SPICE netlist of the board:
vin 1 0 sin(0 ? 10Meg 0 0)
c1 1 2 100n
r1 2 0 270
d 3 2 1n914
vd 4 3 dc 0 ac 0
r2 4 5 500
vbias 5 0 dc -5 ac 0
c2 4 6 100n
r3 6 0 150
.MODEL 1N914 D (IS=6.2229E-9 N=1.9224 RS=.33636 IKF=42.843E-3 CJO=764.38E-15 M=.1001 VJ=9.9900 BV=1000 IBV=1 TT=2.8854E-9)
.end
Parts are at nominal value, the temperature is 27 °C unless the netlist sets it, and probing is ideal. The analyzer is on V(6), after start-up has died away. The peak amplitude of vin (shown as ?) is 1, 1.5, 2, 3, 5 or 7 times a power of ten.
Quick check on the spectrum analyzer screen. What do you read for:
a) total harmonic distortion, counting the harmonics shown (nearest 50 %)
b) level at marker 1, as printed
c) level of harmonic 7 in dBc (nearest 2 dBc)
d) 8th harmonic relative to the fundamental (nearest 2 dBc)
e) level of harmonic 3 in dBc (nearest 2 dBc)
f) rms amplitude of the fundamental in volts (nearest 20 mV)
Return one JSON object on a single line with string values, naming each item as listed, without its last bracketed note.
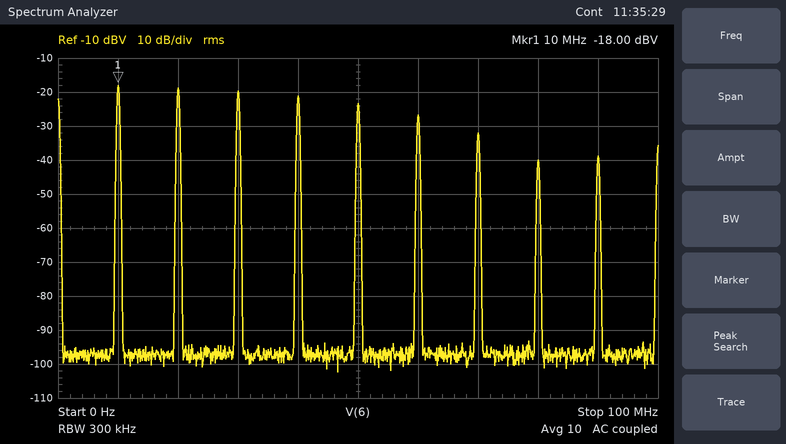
{"total harmonic distortion, counting the harmonics shown": "150 %", "level at marker 1, as printed": "-18.00 dBV", "level of harmonic 7 in dBc": "-14 dBc", "8th harmonic relative to the fundamental": "-22 dBc", "level of harmonic 3 in dBc": "-2 dBc", "rms amplitude of the fundamental in volts": "120 mV"}
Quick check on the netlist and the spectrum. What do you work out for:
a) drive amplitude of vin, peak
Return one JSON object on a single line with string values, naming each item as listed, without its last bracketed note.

{"drive amplitude of vin, peak": "7 V"}
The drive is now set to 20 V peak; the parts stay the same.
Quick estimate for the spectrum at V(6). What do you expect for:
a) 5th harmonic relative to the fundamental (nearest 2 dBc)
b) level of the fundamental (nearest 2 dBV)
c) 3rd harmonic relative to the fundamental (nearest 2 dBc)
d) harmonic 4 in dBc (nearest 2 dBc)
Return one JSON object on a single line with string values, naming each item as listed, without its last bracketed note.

{"5th harmonic relative to the fundamental": "-30 dBc", "level of the fundamental": "4 dBV", "3rd harmonic relative to the fundamental": "-6 dBc", "harmonic 4 in dBc": "-12 dBc"}
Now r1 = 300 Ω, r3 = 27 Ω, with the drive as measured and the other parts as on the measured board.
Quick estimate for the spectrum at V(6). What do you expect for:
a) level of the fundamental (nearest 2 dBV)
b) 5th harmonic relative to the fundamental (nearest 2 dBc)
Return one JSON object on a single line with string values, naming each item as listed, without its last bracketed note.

{"level of the fundamental": "-28 dBV", "5th harmonic relative to the fundamental": "-2 dBc"}
